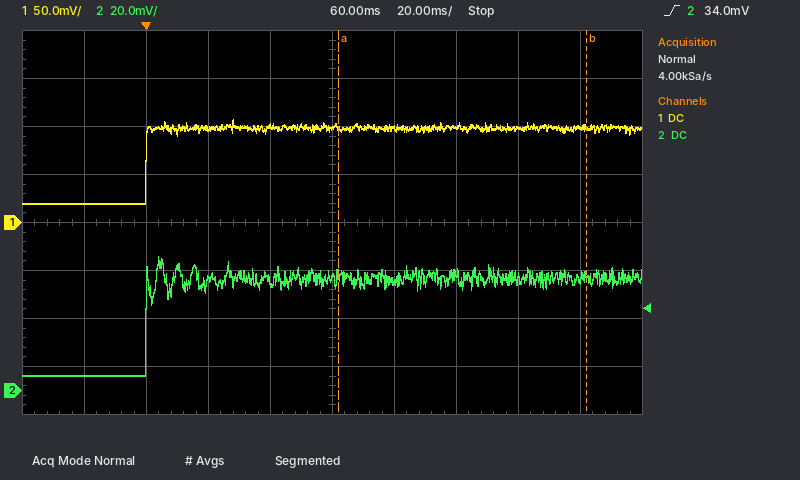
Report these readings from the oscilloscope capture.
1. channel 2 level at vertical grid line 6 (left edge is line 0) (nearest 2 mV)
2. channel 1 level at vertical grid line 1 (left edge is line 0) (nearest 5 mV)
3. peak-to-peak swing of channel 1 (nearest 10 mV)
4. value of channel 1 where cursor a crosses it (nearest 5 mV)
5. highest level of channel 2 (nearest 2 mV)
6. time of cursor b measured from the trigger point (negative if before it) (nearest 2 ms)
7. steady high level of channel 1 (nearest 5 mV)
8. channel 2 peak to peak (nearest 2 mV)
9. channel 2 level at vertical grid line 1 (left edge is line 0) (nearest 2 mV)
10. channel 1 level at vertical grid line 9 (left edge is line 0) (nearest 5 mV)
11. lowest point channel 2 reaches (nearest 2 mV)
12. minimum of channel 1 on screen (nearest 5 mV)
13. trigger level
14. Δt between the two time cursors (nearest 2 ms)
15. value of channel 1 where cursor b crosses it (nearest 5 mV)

46 mV
20 mV
90 mV
100 mV
56 mV
+142 ms
100 mV
50 mV
6 mV
100 mV
6 mV
20 mV
34.0 mV
80 ms
100 mV
